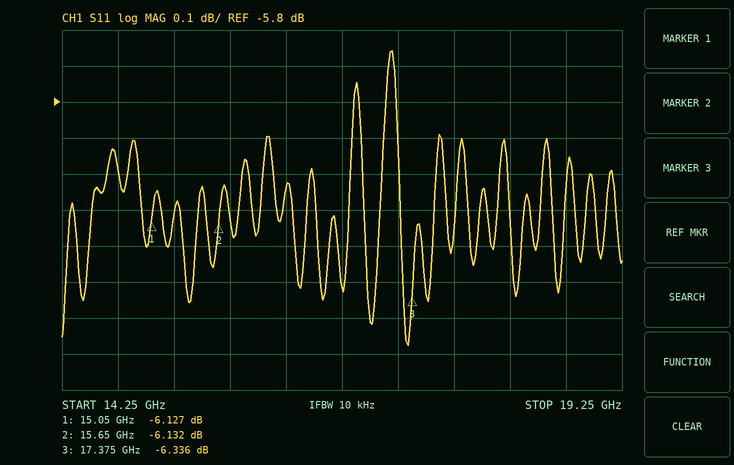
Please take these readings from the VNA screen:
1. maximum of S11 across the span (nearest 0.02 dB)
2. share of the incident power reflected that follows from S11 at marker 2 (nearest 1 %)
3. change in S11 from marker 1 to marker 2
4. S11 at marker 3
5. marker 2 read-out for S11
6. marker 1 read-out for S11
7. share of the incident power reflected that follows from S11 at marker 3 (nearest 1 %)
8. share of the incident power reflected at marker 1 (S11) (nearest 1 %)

-5.66 dB
24 %
-0.005 dB
-6.336 dB
-6.132 dB
-6.127 dB
23 %
24 %
